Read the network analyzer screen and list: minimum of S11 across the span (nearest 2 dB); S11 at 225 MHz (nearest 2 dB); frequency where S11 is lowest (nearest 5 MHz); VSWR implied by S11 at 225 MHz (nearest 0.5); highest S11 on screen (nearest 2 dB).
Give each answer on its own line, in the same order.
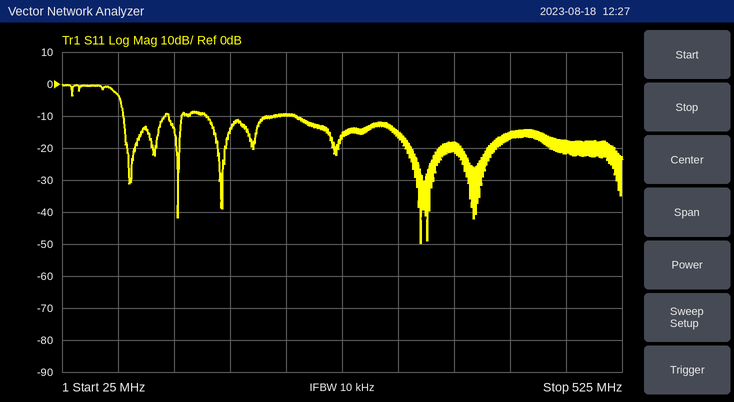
-50 dB
-10 dB
345 MHz
2.0
0 dB
